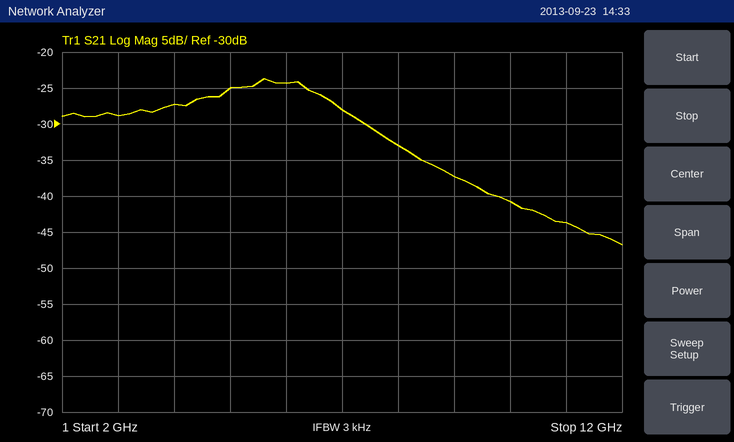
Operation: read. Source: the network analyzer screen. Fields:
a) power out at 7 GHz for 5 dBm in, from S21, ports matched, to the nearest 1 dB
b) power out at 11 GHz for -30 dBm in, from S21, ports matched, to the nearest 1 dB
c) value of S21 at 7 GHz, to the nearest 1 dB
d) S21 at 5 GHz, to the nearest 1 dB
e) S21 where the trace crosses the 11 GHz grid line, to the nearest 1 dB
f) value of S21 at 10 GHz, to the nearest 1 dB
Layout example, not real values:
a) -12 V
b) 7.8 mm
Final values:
a) -23 dBm
b) -74 dBm
c) -28 dB
d) -25 dB
e) -44 dB
f) -41 dB
